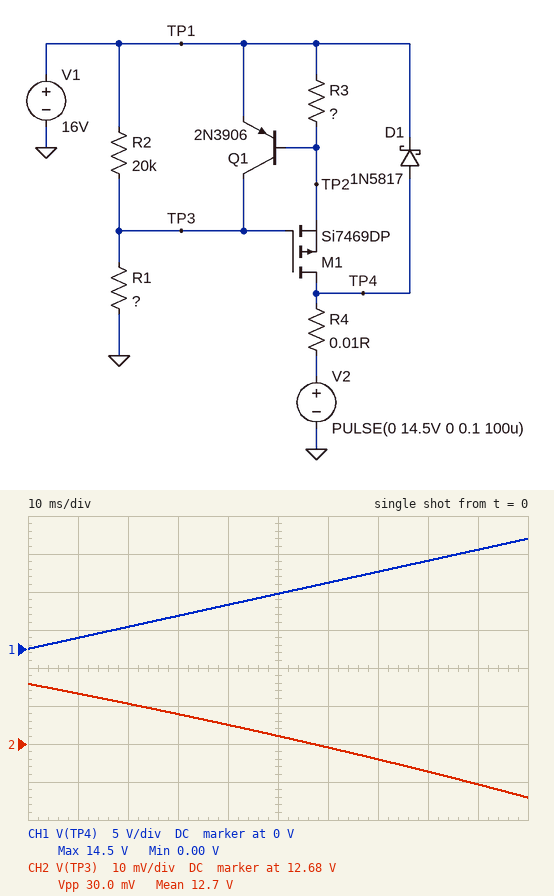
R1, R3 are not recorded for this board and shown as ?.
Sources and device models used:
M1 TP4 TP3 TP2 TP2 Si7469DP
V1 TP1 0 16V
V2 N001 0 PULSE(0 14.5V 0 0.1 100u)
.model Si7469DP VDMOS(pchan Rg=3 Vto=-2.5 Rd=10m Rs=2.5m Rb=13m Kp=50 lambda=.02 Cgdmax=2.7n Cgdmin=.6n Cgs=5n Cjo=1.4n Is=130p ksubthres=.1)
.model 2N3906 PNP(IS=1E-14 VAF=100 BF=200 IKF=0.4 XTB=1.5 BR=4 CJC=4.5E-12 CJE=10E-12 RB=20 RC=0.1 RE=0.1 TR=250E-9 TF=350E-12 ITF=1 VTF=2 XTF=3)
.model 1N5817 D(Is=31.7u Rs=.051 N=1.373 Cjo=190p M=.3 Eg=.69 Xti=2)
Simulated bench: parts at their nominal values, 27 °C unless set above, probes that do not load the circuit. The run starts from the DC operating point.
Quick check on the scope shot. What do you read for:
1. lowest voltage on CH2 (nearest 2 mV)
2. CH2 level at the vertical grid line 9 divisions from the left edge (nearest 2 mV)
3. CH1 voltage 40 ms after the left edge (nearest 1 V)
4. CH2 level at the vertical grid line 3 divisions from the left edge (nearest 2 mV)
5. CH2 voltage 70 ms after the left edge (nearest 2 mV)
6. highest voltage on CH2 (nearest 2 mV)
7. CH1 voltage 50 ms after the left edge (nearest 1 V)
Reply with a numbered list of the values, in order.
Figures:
1. 12.666 V
2. 12.670 V
3. 6 V
4. 12.688 V
5. 12.676 V
6. 12.696 V
7. 7 V
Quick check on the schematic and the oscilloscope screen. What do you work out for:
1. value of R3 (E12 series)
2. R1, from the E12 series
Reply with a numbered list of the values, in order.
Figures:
1. 0.47 Ω
2. 33 kΩ
